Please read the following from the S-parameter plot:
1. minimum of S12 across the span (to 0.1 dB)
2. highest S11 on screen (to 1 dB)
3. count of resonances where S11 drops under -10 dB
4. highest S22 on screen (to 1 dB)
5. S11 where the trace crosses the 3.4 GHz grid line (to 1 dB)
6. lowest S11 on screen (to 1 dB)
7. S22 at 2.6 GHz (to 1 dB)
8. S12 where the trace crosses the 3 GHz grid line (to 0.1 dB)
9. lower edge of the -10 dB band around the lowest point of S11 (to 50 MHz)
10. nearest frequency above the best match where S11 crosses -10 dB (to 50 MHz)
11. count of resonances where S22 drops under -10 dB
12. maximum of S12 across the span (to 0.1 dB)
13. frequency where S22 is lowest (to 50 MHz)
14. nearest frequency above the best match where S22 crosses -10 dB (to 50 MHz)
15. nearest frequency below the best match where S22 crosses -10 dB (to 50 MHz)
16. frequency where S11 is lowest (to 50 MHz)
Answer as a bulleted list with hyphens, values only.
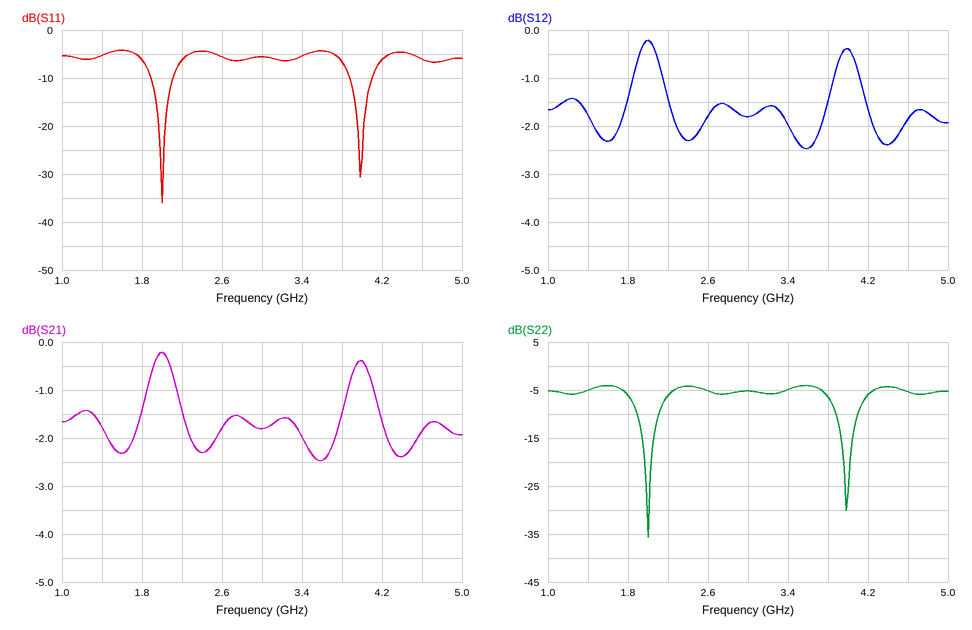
- -2.5 dB
- -4 dB
- 2
- -4 dB
- -5 dB
- -36 dB
- -5 dB
- -1.8 dB
- 1.90 GHz
- 2.10 GHz
- 2
- -0.2 dB
- 2.00 GHz
- 2.10 GHz
- 1.90 GHz
- 2.00 GHz
